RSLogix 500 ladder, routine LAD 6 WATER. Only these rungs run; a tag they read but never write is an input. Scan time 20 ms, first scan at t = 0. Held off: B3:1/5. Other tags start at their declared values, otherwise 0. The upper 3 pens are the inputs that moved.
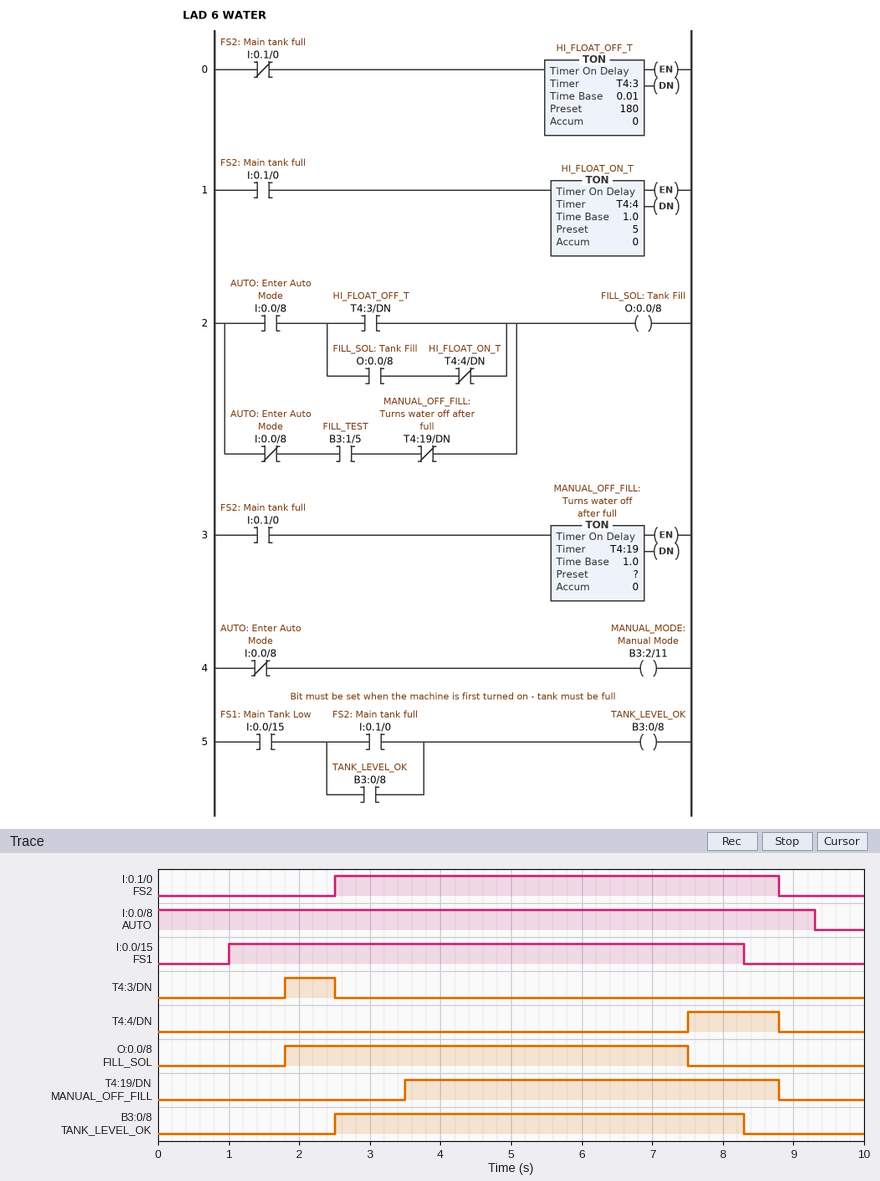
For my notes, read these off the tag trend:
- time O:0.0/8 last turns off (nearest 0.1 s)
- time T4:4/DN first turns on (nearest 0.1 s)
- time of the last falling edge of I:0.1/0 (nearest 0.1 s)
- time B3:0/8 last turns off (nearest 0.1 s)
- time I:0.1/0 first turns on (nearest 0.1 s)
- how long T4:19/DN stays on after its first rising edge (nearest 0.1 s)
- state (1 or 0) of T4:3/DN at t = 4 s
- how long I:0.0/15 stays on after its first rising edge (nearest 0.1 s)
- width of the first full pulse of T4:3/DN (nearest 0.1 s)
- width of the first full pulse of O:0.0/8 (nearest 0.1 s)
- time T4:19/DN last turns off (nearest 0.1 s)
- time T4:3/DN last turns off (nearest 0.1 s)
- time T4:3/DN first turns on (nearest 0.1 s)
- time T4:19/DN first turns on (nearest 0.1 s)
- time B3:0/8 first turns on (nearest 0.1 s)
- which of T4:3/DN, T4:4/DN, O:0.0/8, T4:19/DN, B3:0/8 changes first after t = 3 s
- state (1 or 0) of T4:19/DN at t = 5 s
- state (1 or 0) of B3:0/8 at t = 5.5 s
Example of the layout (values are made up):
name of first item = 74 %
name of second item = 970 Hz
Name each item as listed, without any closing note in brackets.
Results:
time O:0.0/8 last turns off = 7.5 s
time T4:4/DN first turns on = 7.5 s
time of the last falling edge of I:0.1/0 = 8.8 s
time B3:0/8 last turns off = 8.3 s
time I:0.1/0 first turns on = 2.5 s
how long T4:19/DN stays on after its first rising edge = 5.3 s
state (1 or 0) of T4:3/DN at t = 4 s = 0
how long I:0.0/15 stays on after its first rising edge = 7.3 s
width of the first full pulse of T4:3/DN = 0.7 s
width of the first full pulse of O:0.0/8 = 5.7 s
time T4:19/DN last turns off = 8.8 s
time T4:3/DN last turns off = 2.5 s
time T4:3/DN first turns on = 1.8 s
time T4:19/DN first turns on = 3.5 s
time B3:0/8 first turns on = 2.5 s
which of T4:3/DN, T4:4/DN, O:0.0/8, T4:19/DN, B3:0/8 changes first after t = 3 s = T4:19/DN
state (1 or 0) of T4:19/DN at t = 5 s = 1
state (1 or 0) of B3:0/8 at t = 5.5 s = 1
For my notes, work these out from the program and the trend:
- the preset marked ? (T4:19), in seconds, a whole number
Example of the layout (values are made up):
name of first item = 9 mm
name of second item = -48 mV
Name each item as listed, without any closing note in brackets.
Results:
the preset marked ? (T4:19), in seconds, a whole number = 1 s
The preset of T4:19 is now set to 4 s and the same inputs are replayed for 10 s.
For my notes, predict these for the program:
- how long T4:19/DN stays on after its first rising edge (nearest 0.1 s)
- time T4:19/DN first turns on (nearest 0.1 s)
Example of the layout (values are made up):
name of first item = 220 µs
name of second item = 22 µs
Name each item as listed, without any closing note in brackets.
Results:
how long T4:19/DN stays on after its first rising edge = 2.3 s
time T4:19/DN first turns on = 6.5 s
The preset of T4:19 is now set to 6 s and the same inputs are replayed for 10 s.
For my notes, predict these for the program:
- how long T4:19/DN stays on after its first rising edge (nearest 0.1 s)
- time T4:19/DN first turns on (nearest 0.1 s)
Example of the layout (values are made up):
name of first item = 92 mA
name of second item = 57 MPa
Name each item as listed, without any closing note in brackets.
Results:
how long T4:19/DN stays on after its first rising edge = 0.3 s
time T4:19/DN first turns on = 8.5 s
